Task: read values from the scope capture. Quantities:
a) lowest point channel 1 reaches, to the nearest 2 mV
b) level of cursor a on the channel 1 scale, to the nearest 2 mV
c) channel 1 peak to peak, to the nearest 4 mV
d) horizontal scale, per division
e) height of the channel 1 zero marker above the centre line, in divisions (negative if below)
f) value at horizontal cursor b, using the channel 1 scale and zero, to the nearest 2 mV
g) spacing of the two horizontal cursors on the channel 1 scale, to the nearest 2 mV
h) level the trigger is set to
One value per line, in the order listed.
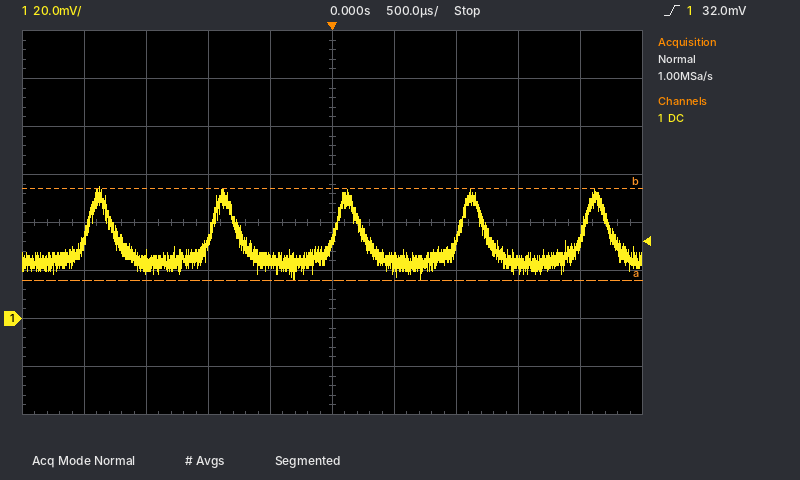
16 mV
16 mV
40 mV
500 µs
-2.0 div
54 mV
38 mV
32.0 mV
